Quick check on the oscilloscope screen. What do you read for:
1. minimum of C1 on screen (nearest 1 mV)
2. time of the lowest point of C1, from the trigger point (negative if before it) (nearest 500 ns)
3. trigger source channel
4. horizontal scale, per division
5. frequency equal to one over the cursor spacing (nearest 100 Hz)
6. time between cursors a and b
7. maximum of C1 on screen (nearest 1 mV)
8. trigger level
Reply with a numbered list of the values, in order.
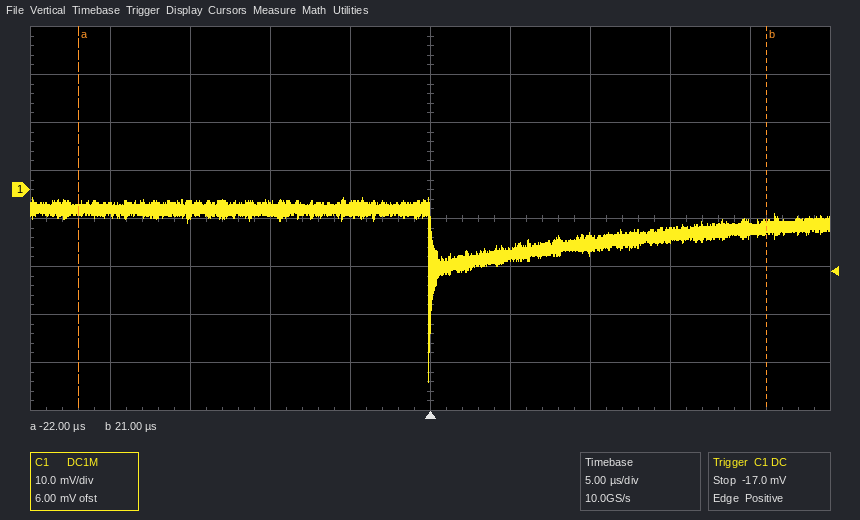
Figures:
1. -40 mV
2. 0.0 µs
3. C1
4. 5 µs
5. 23.3 kHz
6. 43.0 µs
7. -2 mV
8. -17.0 mV
